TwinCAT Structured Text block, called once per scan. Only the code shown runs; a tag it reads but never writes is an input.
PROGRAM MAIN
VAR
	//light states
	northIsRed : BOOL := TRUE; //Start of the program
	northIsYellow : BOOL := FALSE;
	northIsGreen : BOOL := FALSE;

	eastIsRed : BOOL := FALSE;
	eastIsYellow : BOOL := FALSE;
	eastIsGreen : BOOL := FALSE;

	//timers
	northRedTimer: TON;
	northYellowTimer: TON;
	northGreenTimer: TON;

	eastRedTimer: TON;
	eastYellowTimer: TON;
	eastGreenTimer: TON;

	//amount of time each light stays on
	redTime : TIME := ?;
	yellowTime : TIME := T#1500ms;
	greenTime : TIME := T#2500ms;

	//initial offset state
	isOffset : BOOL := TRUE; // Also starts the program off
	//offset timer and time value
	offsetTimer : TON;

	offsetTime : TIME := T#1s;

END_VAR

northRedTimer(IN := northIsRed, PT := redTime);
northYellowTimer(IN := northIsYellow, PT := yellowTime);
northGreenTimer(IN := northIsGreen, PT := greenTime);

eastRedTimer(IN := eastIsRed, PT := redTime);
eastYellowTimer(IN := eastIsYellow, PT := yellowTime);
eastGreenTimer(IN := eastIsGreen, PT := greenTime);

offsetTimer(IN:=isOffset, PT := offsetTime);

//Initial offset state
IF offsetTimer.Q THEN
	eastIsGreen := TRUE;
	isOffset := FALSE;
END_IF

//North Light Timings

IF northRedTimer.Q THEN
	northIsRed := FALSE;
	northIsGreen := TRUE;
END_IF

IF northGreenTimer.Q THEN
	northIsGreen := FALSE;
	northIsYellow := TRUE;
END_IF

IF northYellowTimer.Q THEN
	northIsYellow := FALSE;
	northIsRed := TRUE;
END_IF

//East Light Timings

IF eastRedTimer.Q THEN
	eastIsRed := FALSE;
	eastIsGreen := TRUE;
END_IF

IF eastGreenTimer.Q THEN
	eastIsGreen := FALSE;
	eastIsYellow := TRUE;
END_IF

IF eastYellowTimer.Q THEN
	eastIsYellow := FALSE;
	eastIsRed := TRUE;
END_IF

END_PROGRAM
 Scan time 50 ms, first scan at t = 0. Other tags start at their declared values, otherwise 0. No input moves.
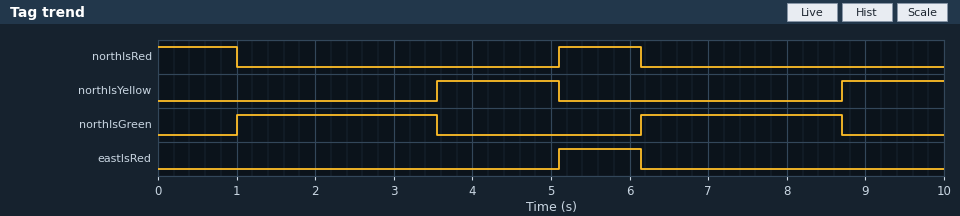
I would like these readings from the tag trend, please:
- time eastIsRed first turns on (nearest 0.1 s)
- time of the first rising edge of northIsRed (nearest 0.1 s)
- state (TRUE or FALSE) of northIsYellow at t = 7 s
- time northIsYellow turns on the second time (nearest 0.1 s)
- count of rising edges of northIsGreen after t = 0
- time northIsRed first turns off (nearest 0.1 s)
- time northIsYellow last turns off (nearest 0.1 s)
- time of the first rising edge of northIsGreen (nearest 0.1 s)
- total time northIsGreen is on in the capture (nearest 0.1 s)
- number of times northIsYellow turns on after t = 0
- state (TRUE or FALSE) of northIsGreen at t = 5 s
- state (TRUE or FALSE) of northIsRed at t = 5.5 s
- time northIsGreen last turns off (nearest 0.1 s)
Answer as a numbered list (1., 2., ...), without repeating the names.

1. 5.1 s
2. 5.1 s
3. FALSE
4. 8.7 s
5. 2
6. 1.0 s
7. 5.1 s
8. 1.0 s
9. 5.1 s
10. 2
11. FALSE
12. TRUE
13. 8.7 s
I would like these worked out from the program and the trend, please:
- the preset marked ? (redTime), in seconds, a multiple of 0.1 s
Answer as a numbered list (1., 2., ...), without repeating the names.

1. 1.0 s
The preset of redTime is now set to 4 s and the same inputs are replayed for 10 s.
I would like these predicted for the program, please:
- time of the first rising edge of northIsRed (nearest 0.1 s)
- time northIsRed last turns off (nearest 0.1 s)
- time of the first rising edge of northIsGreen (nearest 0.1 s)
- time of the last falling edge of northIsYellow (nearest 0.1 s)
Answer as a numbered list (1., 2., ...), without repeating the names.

1. 8.1 s
2. 4.0 s
3. 4.0 s
4. 8.1 s
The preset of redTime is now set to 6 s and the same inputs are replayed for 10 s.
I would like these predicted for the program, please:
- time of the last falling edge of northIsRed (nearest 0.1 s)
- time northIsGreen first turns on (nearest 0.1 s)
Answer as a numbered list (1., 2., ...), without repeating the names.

1. 6.0 s
2. 6.0 s
